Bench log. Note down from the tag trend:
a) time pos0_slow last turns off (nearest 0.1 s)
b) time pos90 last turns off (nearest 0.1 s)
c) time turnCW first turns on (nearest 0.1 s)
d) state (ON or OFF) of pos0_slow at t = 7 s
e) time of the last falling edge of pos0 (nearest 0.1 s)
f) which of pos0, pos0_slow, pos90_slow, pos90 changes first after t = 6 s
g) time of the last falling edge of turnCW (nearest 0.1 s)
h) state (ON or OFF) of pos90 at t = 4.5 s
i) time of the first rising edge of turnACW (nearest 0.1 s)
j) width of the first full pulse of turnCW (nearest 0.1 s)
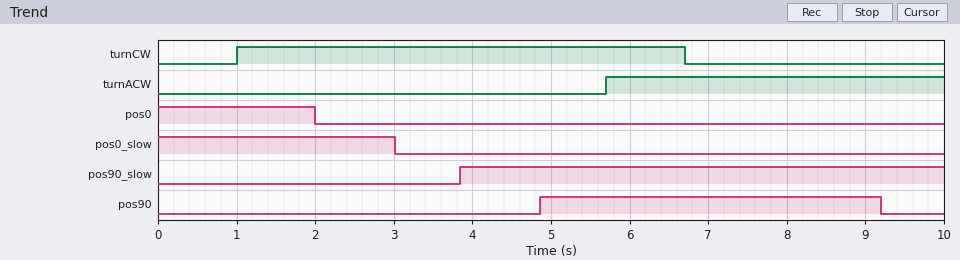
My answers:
3.0 s
9.2 s
1.0 s
OFF
2.0 s
pos90
6.7 s
OFF
5.7 s
5.7 s
